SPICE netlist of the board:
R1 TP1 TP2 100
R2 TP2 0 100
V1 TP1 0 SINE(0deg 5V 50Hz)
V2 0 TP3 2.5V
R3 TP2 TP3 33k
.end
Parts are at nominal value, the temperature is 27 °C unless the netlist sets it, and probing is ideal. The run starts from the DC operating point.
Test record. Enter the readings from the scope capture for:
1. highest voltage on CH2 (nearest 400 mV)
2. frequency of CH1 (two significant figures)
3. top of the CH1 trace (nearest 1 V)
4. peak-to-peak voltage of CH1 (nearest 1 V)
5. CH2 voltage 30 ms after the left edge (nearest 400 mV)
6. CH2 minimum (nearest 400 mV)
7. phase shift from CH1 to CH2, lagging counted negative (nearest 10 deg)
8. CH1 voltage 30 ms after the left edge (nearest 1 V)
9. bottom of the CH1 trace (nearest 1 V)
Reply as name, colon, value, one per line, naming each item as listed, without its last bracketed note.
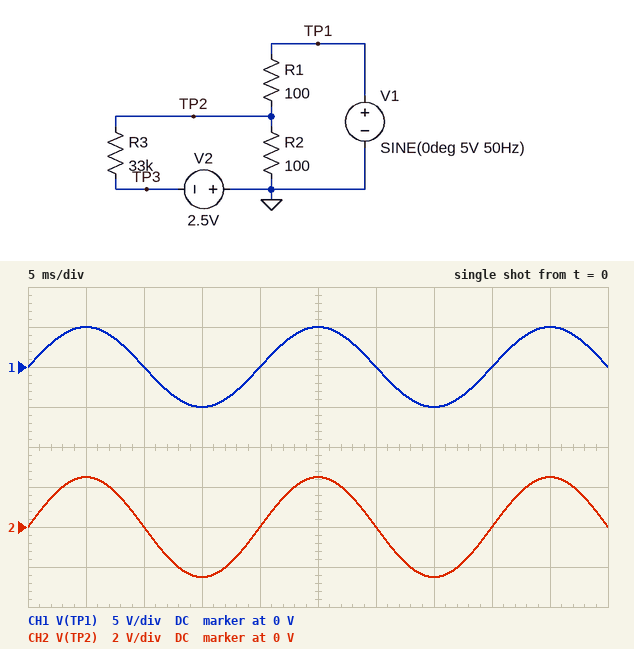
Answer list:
highest voltage on CH2: 2.4 V
frequency of CH1: 50 Hz
top of the CH1 trace: 5 V
peak-to-peak voltage of CH1: 10 V
CH2 voltage 30 ms after the left edge: 0 V
CH2 minimum: -2.4 V
phase shift from CH1 to CH2, lagging counted negative: 0 deg
CH1 voltage 30 ms after the left edge: 0 V
bottom of the CH1 trace: -5 V
